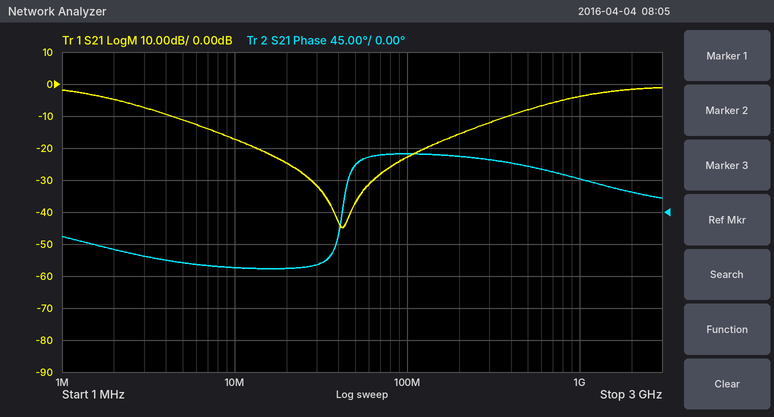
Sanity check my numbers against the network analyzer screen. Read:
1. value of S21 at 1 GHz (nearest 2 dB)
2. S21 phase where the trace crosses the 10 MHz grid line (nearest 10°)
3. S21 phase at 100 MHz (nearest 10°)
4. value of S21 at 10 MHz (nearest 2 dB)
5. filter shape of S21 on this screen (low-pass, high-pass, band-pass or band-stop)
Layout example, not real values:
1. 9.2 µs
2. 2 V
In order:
1. -4 dB
2. -80°
3. 80°
4. -18 dB
5. band-stop
